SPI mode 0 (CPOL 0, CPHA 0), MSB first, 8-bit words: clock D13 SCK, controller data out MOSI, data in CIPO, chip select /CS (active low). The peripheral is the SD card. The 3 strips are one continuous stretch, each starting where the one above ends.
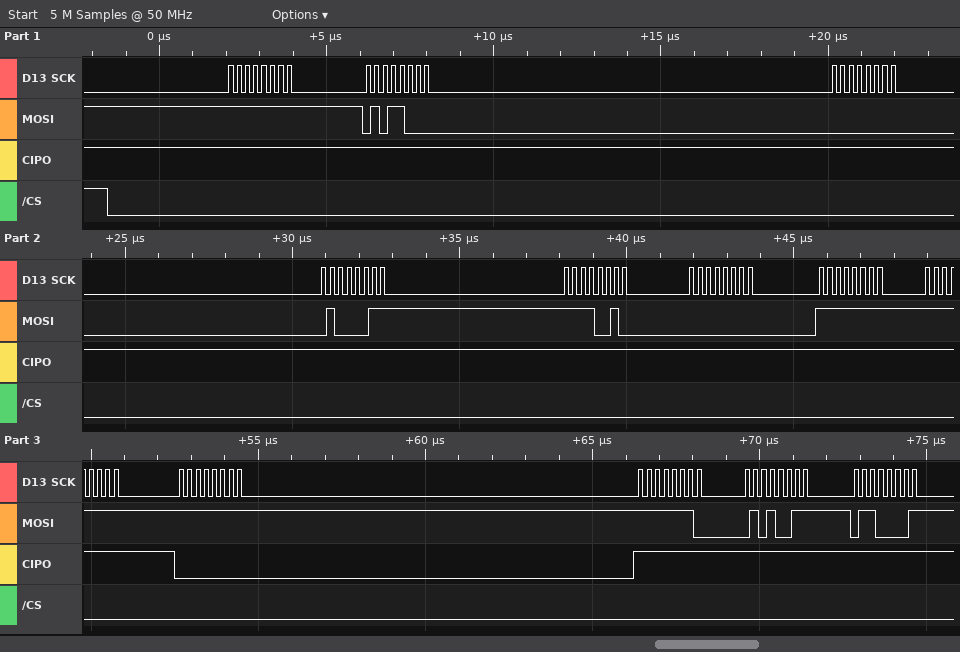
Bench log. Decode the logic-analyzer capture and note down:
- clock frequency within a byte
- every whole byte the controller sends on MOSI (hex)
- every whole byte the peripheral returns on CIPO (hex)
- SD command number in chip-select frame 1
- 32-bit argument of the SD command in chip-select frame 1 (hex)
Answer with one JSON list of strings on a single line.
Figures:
["4 MHz", "FF 58 00 43 F2 00 FF FF FF FE 53 61", "FF FF FF FF FF FF FF FF 00 FF FF FF", "CMD24", "0x0043F200"]
